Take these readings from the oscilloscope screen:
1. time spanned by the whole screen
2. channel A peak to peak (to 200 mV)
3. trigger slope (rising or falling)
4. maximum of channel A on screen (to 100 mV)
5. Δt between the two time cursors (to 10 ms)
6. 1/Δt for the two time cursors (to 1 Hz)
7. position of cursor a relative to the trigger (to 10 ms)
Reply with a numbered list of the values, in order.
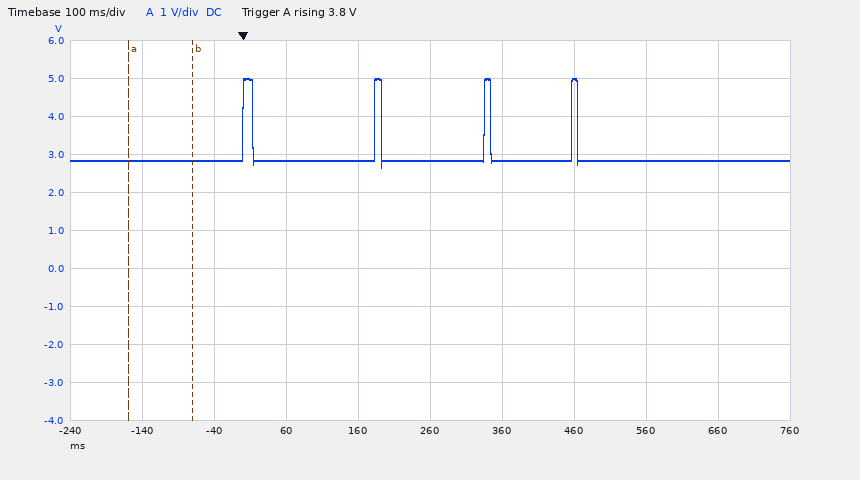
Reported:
1. 1 s
2. 2.4 V
3. rising
4. 5.0 V
5. 90 ms
6. 11 Hz
7. -160 ms
